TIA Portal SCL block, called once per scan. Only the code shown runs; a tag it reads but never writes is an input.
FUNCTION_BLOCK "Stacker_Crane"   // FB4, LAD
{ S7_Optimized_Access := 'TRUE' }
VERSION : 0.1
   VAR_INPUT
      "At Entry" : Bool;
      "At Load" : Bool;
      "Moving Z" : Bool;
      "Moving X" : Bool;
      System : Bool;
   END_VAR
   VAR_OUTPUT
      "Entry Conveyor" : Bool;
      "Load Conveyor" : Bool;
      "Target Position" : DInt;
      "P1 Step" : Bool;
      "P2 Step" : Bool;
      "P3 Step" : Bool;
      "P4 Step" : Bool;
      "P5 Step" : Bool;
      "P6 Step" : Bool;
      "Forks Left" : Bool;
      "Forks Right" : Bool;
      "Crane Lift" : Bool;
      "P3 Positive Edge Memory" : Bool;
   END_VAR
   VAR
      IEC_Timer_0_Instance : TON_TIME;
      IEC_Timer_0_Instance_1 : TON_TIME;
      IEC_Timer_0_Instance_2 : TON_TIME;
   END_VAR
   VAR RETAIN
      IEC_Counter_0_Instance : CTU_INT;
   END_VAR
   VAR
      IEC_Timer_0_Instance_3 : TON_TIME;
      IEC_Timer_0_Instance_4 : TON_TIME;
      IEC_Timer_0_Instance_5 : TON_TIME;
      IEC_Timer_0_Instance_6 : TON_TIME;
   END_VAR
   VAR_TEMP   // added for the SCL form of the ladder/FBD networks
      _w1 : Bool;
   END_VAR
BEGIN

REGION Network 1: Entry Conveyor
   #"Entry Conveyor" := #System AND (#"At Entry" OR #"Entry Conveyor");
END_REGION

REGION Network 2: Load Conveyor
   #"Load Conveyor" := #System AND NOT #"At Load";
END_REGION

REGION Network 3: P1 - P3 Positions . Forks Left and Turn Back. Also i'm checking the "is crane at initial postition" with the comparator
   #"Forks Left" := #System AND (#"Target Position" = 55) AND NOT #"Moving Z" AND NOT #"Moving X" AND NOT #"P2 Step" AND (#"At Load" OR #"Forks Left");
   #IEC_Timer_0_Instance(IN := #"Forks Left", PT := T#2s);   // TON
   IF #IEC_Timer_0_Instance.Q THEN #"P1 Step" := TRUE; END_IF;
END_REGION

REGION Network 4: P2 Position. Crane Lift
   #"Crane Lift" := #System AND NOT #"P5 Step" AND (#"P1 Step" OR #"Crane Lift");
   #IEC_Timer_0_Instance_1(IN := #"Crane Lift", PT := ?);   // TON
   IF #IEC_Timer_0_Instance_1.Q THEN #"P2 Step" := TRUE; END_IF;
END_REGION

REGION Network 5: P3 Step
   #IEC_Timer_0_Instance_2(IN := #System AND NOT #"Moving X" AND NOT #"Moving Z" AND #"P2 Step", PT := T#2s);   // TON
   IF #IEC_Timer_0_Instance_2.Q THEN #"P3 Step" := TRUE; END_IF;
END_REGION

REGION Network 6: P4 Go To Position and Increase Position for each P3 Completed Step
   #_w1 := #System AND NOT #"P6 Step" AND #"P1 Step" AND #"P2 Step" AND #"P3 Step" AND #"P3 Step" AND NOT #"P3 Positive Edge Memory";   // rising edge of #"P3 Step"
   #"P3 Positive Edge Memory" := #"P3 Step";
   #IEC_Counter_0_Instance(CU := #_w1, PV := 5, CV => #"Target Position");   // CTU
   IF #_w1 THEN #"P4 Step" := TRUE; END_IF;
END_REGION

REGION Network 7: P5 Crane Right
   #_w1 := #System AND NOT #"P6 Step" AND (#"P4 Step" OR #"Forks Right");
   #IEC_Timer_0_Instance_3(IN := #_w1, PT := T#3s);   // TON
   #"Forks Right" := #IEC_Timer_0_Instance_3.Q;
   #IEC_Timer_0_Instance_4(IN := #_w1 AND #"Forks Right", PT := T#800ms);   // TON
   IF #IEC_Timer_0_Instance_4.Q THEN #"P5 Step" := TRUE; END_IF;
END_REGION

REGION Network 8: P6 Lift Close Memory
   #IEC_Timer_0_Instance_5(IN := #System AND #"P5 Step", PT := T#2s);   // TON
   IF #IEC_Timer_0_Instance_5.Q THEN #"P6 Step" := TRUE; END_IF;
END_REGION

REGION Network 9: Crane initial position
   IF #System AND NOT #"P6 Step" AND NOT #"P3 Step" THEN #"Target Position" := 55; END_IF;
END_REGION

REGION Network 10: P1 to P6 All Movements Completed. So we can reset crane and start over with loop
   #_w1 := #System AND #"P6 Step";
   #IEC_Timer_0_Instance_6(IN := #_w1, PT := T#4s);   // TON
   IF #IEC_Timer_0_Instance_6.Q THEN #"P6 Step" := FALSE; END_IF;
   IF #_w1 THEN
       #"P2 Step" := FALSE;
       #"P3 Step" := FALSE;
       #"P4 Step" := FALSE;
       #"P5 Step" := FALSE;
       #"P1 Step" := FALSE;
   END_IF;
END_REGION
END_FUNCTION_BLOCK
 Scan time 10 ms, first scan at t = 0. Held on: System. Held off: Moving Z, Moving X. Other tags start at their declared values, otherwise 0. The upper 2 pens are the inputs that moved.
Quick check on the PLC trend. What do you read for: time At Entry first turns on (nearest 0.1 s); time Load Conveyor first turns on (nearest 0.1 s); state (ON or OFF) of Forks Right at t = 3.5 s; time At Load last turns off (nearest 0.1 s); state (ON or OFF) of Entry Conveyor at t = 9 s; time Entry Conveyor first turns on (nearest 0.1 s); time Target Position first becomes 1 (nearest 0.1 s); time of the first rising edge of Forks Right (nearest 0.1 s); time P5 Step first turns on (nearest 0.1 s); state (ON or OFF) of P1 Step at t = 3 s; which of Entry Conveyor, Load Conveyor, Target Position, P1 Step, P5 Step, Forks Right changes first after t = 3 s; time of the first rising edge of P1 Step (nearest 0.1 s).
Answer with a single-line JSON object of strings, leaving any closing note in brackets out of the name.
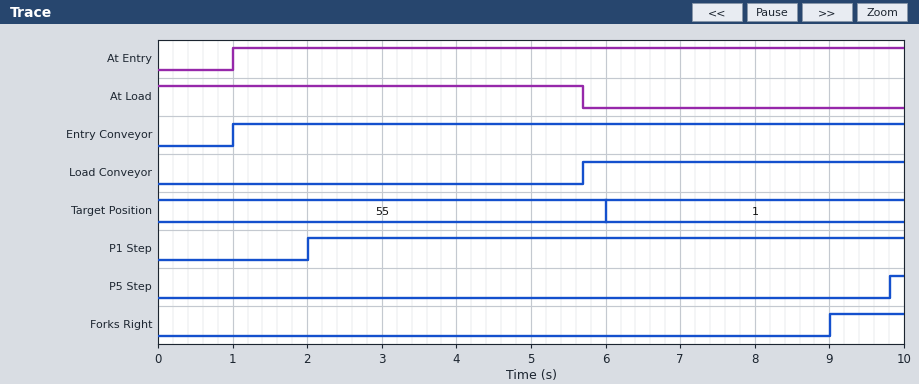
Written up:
{"time At Entry first turns on": "1.0 s", "time Load Conveyor first turns on": "5.7 s", "state (ON or OFF) of Forks Right at t = 3.5 s": "OFF", "time At Load last turns off": "5.7 s", "state (ON or OFF) of Entry Conveyor at t = 9 s": "ON", "time Entry Conveyor first turns on": "1.0 s", "time Target Position first becomes 1": "6.0 s", "time of the first rising edge of Forks Right": "9.0 s", "time P5 Step first turns on": "9.8 s", "state (ON or OFF) of P1 Step at t = 3 s": "ON", "which of Entry Conveyor, Load Conveyor, Target Position, P1 Step, P5 Step, Forks Right changes first after t = 3 s": "Load Conveyor", "time of the first rising edge of P1 Step": "2.0 s"}
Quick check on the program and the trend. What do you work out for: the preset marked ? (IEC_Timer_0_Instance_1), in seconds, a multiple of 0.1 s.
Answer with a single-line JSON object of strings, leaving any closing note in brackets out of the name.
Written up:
{"the preset marked ? (IEC_Timer_0_Instance_1), in seconds, a multiple of 0.1 s": "2.0 s"}
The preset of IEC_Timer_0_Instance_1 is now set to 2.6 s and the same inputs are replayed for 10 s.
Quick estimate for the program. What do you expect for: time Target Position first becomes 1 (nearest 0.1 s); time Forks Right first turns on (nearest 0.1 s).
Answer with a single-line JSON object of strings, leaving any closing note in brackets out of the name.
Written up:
{"time Target Position first becomes 1": "6.6 s", "time Forks Right first turns on": "9.6 s"}
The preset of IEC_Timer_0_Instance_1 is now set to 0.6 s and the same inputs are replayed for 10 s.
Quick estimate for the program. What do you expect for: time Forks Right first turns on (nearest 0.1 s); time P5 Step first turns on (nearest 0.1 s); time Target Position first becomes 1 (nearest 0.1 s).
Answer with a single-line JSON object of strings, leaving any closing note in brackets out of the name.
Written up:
{"time Forks Right first turns on": "7.6 s", "time P5 Step first turns on": "8.4 s", "time Target Position first becomes 1": "4.6 s"}
